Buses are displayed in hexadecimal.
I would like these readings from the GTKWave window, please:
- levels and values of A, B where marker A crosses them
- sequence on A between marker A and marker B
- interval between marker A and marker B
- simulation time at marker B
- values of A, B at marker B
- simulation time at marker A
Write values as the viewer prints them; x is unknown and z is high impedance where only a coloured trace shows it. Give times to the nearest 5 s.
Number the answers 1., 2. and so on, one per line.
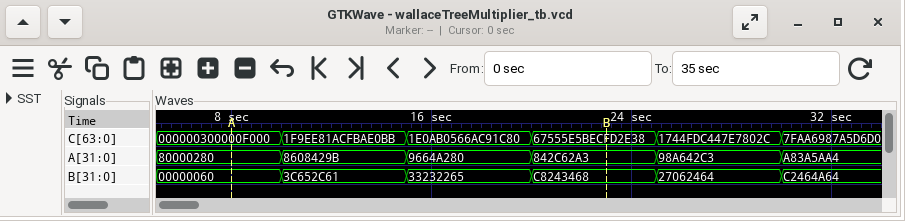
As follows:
1. A=80000280, B=00000060
2. 80000280, 8608429B, 9664A280, 842C62A3
3. 15 s
4. 25 s
5. A=842C62A3, B=C8243468
6. 10 s
